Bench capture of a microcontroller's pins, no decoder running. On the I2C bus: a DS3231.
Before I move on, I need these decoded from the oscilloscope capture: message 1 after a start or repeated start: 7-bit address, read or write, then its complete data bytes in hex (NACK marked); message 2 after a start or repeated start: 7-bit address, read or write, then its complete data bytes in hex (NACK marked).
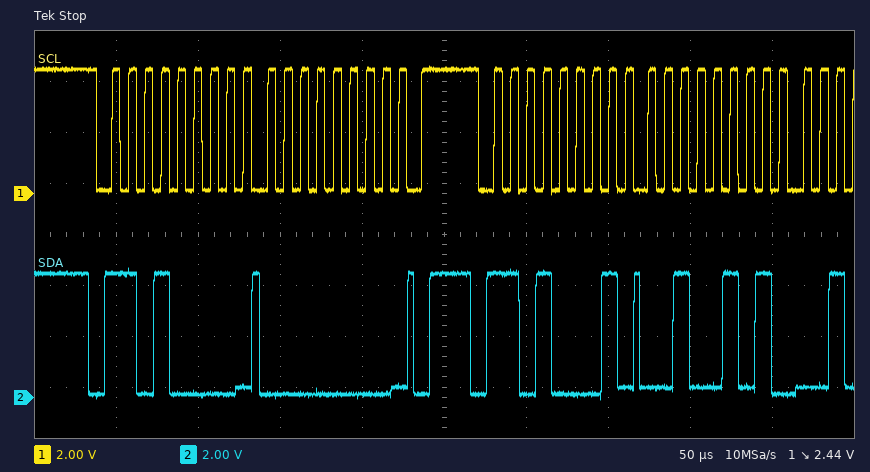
0x68 write: 00
0x68 read: 25
